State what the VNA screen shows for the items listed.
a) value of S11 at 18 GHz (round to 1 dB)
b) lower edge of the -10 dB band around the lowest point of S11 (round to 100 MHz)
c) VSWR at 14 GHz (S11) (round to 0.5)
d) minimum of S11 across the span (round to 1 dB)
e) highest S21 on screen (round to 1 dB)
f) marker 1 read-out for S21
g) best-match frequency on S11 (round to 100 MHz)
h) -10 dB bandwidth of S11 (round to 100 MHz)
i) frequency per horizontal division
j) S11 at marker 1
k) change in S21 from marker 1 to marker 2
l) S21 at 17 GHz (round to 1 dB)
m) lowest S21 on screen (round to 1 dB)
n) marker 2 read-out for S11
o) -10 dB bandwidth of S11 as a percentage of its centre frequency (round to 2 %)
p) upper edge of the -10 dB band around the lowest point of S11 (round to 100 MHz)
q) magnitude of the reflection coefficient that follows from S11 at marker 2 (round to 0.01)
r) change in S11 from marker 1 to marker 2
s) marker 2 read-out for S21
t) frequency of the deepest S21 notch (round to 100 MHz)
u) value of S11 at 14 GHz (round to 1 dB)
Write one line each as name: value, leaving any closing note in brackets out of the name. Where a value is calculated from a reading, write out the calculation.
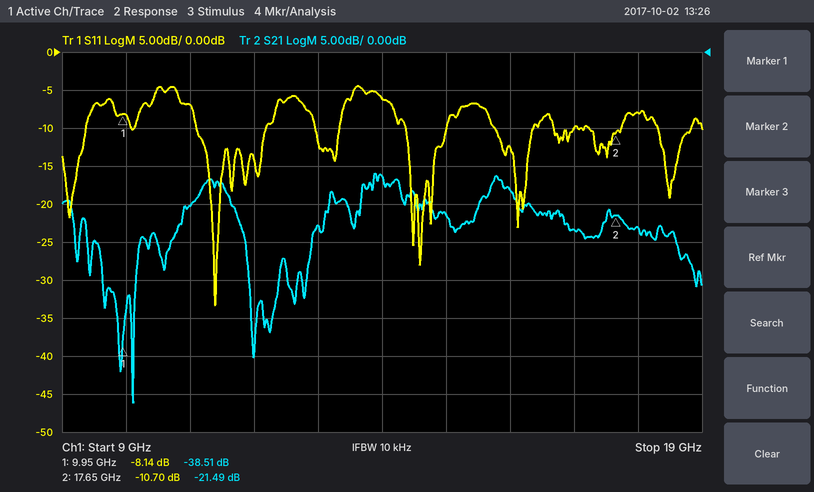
value of S11 at 18 GHz: -8 dB
lower edge of the -10 dB band around the lowest point of S11: 11.1 GHz
VSWR at 14 GHz (S11): |Γ| = 10^(-6/20) = 0.5012; VSWR = (1 + 0.5012)/(1 − 0.5012) ≈ 3.0
minimum of S11 across the span: -33 dB
highest S21 on screen: -16 dB
marker 1 read-out for S21: -38.51 dB
best-match frequency on S11: 11.4 GHz
-10 dB bandwidth of S11: 12.2 GHz − 11.1 GHz = 1.1 GHz
frequency per horizontal division: 1 GHz
S11 at marker 1: -8.14 dB
change in S21 from marker 1 to marker 2: -21.49 − (-38.51) = 17.02 dB
S21 at 17 GHz: -23 dB
lowest S21 on screen: -46 dB
marker 2 read-out for S11: -10.70 dB
-10 dB bandwidth of S11 as a percentage of its centre frequency: 1.1 GHz / 11.65 GHz ≈ 9.44 %, so 10 % to the nearest 2 %
upper edge of the -10 dB band around the lowest point of S11: 12.2 GHz
magnitude of the reflection coefficient that follows from S11 at marker 2: 10^(-10.7/20) ≈ 0.29
change in S11 from marker 1 to marker 2: -10.7 − (-8.14) = -2.56 dB
marker 2 read-out for S21: -21.49 dB
frequency of the deepest S21 notch: 10.1 GHz
value of S11 at 14 GHz: -6 dB
